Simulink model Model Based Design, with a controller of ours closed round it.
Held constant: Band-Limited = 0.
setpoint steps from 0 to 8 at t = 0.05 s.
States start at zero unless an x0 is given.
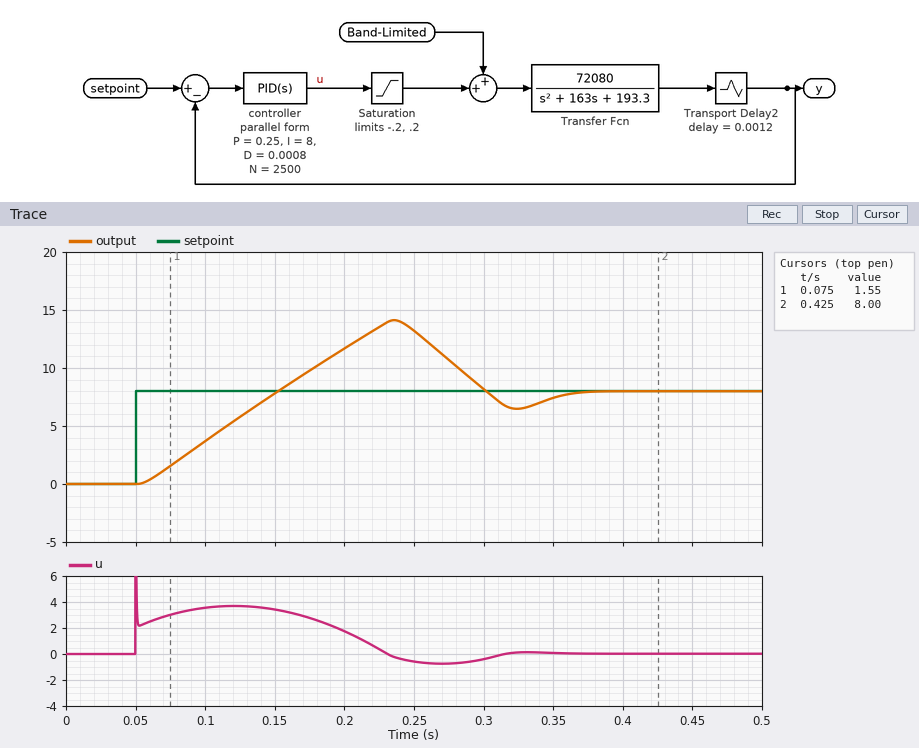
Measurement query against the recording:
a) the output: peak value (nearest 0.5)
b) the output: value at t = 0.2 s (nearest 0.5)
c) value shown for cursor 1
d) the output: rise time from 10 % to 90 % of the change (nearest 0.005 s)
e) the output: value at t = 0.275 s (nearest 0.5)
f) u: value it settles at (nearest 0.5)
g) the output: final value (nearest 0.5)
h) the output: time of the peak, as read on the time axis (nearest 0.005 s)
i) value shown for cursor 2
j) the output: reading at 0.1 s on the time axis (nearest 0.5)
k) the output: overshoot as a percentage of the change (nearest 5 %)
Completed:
14.0
11.5
1.55
0.075 s
10.5
0.0
8.0
0.235 s
8.00
3.5
75 %
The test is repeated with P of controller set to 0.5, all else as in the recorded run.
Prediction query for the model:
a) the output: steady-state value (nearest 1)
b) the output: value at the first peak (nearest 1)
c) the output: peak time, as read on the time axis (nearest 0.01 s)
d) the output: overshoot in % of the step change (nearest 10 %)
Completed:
8
13
0.22 s
60 %
